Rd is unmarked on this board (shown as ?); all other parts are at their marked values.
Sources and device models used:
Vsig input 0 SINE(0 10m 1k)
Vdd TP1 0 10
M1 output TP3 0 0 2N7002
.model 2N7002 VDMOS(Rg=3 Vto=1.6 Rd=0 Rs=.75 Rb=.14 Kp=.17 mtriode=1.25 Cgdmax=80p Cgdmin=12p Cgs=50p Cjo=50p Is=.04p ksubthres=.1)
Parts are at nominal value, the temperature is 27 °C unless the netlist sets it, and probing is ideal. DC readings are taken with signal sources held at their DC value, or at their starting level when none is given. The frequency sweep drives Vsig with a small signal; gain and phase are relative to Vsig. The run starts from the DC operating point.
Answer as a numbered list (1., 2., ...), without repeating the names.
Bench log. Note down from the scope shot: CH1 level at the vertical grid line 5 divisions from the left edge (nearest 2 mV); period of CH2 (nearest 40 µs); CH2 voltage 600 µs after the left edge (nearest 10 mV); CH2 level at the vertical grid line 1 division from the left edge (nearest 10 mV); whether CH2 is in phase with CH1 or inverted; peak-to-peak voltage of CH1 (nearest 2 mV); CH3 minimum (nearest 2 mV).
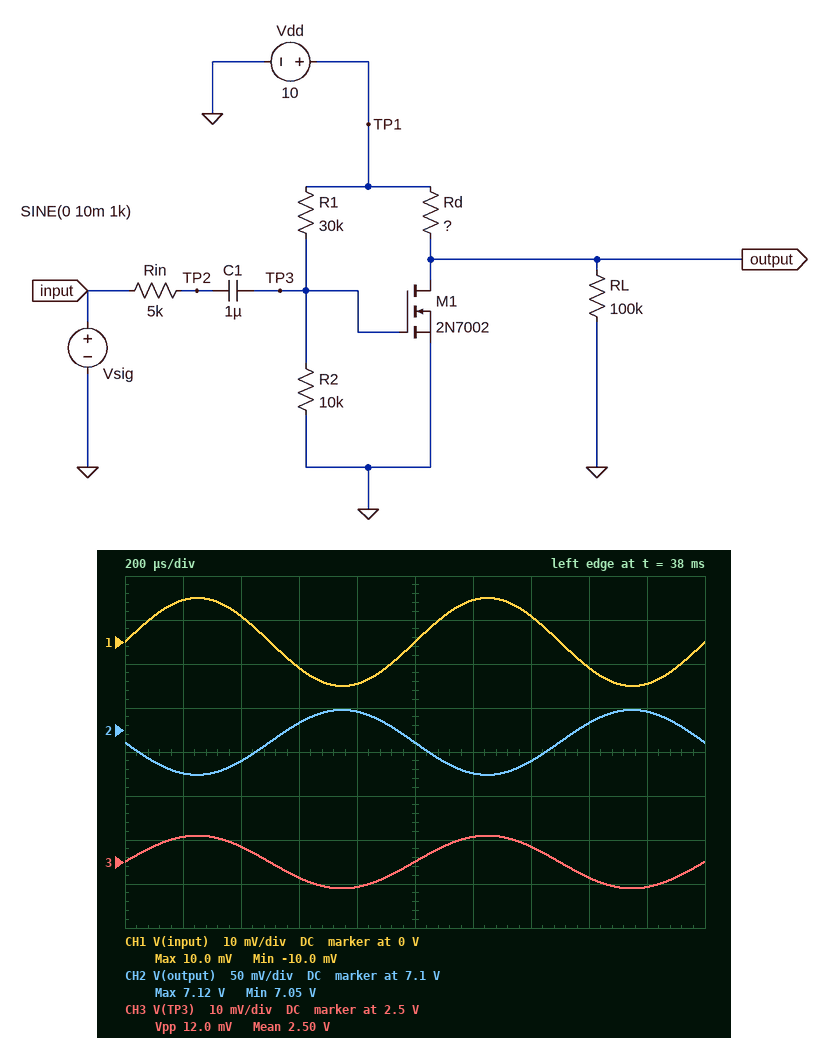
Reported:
1. 0 V
2. 1.00 ms
3. 7.11 V
4. 7.05 V
5. inverted
6. 20 mV
7. 2.494 V
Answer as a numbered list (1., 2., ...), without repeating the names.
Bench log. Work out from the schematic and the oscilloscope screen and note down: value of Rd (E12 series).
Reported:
1. 47 Ω
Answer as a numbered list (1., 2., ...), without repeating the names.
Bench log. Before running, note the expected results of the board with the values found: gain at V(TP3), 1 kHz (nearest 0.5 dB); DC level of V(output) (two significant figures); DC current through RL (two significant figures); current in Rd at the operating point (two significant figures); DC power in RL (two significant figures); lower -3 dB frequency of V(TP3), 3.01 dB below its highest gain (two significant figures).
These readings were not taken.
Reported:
1. -4.5 dB
2. 7.1 V
3. 71 µA
4. 62 mA
5. 500 µW
6. 13 Hz
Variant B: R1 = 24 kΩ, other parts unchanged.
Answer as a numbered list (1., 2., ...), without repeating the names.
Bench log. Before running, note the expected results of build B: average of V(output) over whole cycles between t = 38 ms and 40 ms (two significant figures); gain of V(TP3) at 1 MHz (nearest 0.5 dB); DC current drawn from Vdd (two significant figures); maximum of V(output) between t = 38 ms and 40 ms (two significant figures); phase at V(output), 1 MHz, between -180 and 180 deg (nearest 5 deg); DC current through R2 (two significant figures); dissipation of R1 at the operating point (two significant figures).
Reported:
1. 3.8 V
2. -21.5 dB
3. 130 mA
4. 3.9 V
5. 100 deg
6. 290 µA
7. 2.1 mW
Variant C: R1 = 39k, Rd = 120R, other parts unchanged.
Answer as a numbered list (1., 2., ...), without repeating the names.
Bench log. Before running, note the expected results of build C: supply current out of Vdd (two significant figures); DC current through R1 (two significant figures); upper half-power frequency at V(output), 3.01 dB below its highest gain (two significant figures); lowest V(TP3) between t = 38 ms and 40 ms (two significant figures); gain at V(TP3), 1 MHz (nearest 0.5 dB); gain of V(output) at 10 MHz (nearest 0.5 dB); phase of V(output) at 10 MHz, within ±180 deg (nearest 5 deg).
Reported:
1. 16 mA
2. 200 µA
3. 260 kHz
4. 2.0 V
5. -16.0 dB
6. -17.5 dB
7. 85 deg
